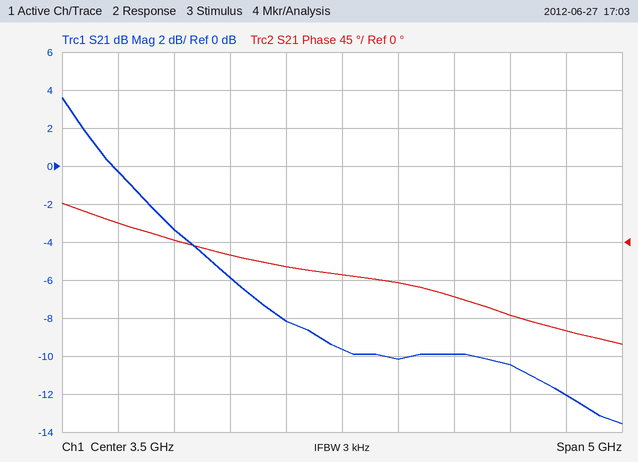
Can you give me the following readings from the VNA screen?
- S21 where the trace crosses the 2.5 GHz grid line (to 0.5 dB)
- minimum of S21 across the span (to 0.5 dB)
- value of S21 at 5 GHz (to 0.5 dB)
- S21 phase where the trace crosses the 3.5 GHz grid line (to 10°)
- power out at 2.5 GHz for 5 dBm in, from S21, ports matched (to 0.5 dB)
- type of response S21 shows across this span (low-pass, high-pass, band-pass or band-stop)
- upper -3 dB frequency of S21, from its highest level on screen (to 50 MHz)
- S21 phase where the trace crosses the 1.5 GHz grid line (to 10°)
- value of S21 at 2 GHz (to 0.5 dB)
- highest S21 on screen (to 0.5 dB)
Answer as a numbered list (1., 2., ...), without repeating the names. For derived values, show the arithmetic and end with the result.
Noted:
1. -6.0 dB
2. -13.5 dB
3. -10.5 dB
4. -40°
5. 5 dBm + (-6.0 dB) = -1.0 dBm
6. low-pass
7. 1.35 GHz
8. 20°
9. -3.5 dB
10. 3.5 dB
